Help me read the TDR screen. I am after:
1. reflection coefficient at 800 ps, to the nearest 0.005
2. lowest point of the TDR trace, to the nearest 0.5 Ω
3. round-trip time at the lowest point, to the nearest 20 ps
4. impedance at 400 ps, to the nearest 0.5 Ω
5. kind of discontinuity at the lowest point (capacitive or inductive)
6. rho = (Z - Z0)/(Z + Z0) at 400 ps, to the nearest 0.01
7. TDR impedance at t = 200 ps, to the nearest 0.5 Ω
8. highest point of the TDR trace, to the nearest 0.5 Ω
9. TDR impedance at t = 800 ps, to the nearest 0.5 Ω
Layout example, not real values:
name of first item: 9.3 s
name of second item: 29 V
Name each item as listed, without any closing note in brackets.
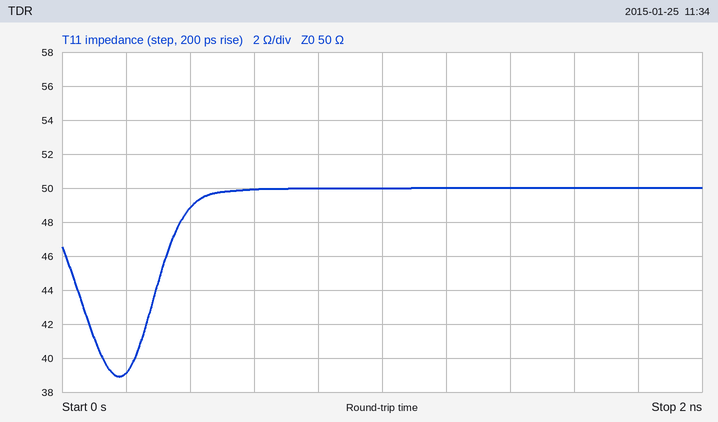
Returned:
reflection coefficient at 800 ps, to the nearest 0.005: 0.000
lowest point of the TDR trace, to the nearest 0.5 Ω: 39.0 Ω
round-trip time at the lowest point, to the nearest 20 ps: 180 ps
impedance at 400 ps, to the nearest 0.5 Ω: 49.0 Ω
kind of discontinuity at the lowest point: capacitive
rho = (Z - Z0)/(Z + Z0) at 400 ps, to the nearest 0.01: -0.01
TDR impedance at t = 200 ps, to the nearest 0.5 Ω: 39.0 Ω
highest point of the TDR trace, to the nearest 0.5 Ω: 50.0 Ω
TDR impedance at t = 800 ps, to the nearest 0.5 Ω: 50.0 Ω
